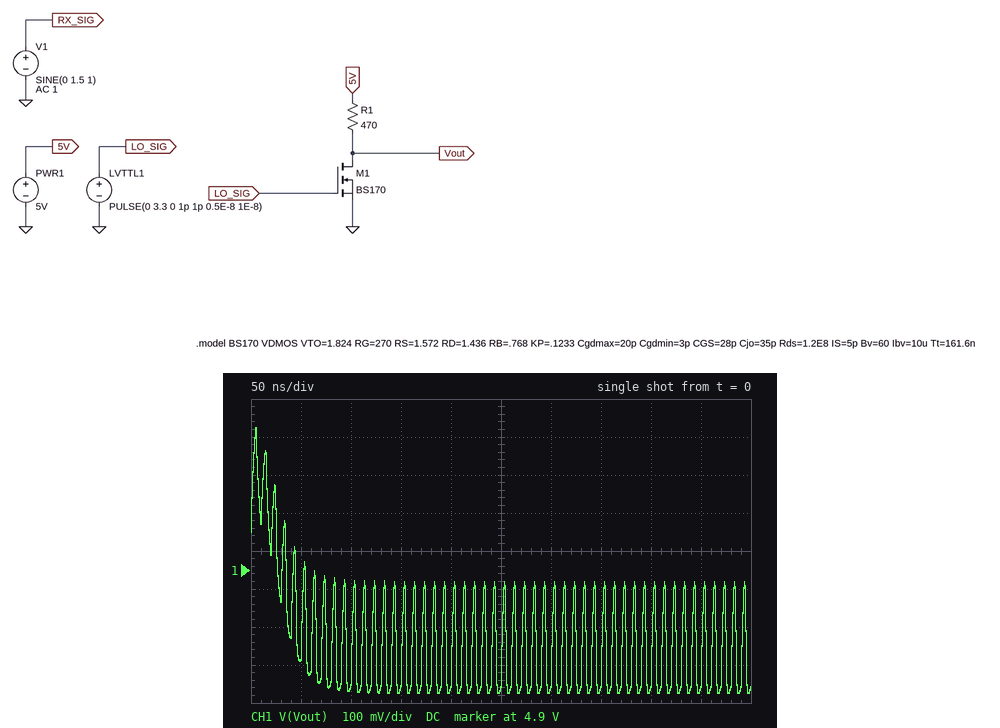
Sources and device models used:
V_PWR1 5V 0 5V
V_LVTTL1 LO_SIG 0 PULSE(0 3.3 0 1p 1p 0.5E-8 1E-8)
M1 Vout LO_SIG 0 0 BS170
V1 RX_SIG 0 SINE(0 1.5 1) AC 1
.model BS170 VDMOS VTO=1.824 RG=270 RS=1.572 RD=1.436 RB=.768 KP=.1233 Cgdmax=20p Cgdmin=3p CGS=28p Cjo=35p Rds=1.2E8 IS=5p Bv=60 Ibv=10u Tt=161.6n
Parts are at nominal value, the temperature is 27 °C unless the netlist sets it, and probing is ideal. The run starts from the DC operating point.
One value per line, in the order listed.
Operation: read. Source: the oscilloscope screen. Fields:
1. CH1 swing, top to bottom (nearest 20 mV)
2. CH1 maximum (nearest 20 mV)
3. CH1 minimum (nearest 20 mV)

700 mV
5.28 V
4.58 V
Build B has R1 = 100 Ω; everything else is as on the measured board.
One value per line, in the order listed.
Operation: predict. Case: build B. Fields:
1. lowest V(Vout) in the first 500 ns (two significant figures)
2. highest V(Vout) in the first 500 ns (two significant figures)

4.8 V
5.1 V
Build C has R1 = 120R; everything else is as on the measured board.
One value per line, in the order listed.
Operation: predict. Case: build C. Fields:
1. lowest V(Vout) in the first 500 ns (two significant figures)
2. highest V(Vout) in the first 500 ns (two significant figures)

4.8 V
5.1 V
